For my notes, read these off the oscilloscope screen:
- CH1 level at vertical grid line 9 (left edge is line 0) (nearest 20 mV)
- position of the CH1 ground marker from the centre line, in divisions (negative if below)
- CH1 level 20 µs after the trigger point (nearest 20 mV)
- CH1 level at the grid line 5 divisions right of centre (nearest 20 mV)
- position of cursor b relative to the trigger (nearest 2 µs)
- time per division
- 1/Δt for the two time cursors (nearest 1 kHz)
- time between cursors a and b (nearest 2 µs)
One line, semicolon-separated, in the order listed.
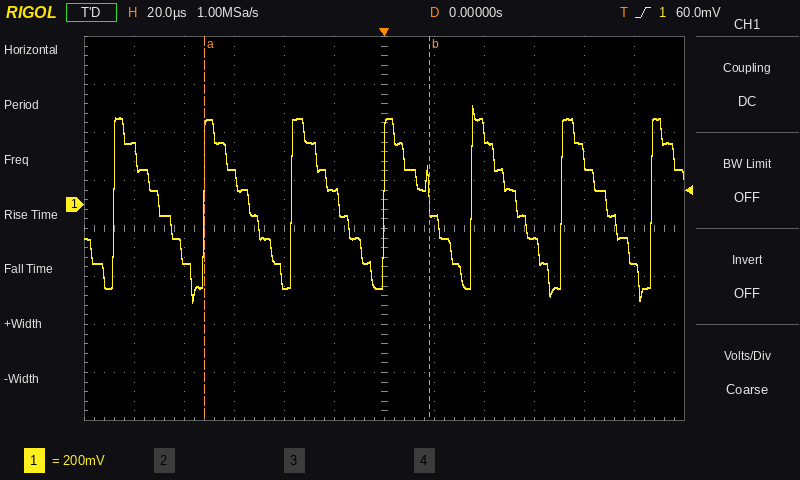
-140 mV; +0.5 div; -40 mV; -240 mV; +18 µs; 20 µs; 11 kHz; 90 µs
